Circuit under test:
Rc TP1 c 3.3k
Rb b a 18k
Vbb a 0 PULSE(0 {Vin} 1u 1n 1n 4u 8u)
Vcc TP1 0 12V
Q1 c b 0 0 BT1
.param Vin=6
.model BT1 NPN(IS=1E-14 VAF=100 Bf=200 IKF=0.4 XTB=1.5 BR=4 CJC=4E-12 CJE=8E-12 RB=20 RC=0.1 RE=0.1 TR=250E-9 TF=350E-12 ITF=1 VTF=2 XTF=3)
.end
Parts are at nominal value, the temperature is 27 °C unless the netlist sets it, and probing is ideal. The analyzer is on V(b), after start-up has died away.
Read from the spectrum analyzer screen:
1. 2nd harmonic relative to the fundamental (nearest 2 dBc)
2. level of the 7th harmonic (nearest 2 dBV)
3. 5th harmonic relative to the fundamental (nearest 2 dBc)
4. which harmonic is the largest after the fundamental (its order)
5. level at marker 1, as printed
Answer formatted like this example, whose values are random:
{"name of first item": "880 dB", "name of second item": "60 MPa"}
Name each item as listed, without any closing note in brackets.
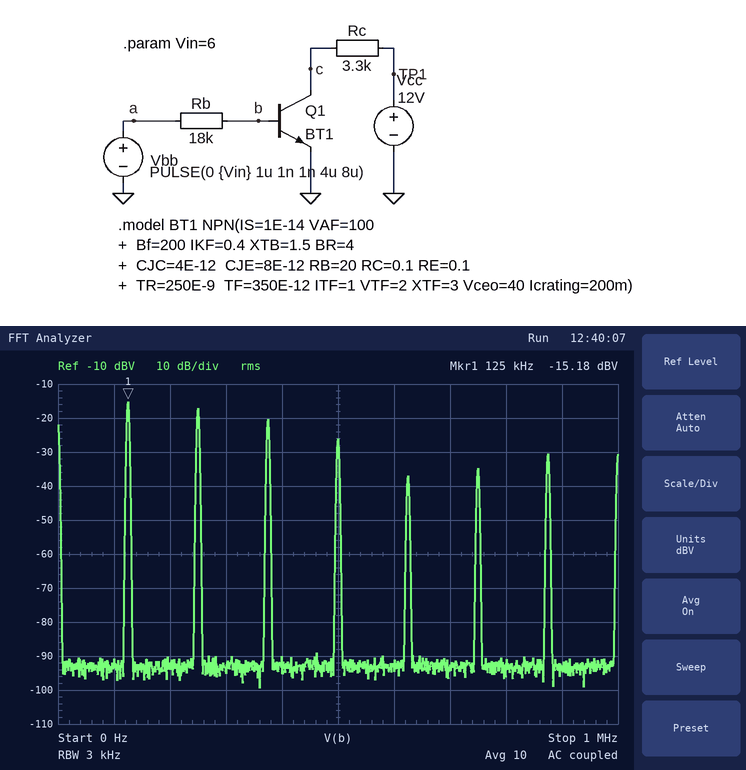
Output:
{"2nd harmonic relative to the fundamental": "-2 dBc", "level of the 7th harmonic": "-30 dBV", "5th harmonic relative to the fundamental": "-22 dBc", "which harmonic is the largest after the fundamental": "2", "level at marker 1, as printed": "-15.18 dBV"}
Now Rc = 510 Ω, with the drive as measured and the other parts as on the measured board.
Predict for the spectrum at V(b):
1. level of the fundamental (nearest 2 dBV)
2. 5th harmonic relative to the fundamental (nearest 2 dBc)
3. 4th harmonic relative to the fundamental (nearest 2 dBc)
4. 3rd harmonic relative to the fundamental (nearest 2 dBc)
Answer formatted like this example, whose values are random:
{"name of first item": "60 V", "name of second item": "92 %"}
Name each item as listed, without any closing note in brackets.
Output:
{"level of the fundamental": "-10 dBV", "5th harmonic relative to the fundamental": "-16 dBc", "4th harmonic relative to the fundamental": "-12 dBc", "3rd harmonic relative to the fundamental": "-26 dBc"}
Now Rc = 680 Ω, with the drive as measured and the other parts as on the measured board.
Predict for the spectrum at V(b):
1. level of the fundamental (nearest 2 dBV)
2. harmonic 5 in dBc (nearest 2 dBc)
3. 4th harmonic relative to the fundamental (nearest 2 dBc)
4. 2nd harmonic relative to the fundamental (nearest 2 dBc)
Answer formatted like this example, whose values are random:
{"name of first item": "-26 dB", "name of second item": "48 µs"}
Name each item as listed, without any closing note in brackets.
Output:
{"level of the fundamental": "-12 dBV", "harmonic 5 in dBc": "-14 dBc", "4th harmonic relative to the fundamental": "-14 dBc", "2nd harmonic relative to the fundamental": "-6 dBc"}
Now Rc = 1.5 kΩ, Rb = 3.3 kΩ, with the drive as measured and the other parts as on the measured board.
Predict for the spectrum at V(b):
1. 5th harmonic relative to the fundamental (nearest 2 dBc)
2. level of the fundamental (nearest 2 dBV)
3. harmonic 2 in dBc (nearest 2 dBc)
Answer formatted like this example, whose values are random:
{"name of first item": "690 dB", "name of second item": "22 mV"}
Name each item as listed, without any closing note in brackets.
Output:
{"5th harmonic relative to the fundamental": "-16 dBc", "level of the fundamental": "-12 dBV", "harmonic 2 in dBc": "-4 dBc"}
